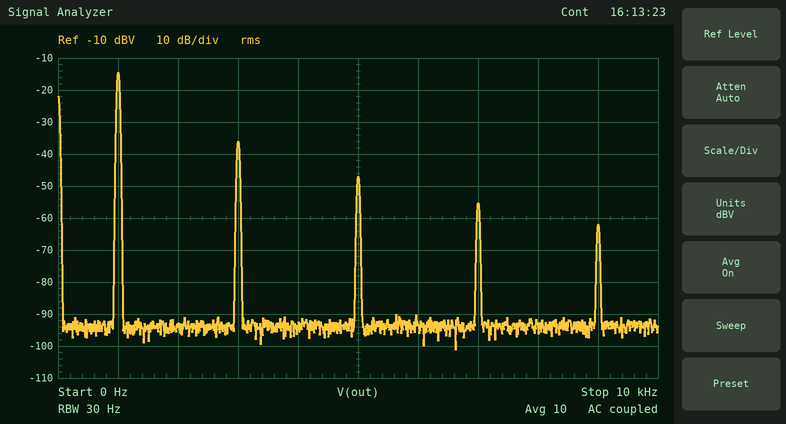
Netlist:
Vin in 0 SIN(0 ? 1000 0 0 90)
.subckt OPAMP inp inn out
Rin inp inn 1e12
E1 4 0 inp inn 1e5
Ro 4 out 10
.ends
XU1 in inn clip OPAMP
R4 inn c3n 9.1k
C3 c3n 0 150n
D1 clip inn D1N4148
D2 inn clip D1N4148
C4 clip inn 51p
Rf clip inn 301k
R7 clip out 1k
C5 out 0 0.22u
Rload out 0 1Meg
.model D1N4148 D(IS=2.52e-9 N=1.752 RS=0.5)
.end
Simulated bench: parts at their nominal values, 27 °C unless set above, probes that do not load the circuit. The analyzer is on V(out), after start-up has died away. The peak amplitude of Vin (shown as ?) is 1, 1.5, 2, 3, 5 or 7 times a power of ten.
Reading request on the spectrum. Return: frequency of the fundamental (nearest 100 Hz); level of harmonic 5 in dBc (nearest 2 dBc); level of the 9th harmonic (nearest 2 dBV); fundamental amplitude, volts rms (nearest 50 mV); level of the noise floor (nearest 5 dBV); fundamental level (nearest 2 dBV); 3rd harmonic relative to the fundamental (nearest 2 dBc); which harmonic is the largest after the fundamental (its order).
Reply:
1.0 kHz
-32 dBc
-62 dBV
200 mV
-95 dBV
-14 dBV
-22 dBc
3
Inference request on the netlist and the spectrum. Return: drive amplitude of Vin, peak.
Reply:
50 mV
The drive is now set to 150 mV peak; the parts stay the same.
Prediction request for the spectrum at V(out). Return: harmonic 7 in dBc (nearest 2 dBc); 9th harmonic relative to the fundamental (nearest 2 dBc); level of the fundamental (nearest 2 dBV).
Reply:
-38 dBc
-44 dBc
-12 dBV
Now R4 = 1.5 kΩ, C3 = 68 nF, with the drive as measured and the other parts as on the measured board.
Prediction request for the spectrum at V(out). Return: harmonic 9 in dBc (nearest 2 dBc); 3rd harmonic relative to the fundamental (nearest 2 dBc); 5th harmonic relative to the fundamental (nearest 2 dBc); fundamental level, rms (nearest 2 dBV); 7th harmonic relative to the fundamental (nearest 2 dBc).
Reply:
-42 dBc
-20 dBc
-30 dBc
-14 dBV
-36 dBc
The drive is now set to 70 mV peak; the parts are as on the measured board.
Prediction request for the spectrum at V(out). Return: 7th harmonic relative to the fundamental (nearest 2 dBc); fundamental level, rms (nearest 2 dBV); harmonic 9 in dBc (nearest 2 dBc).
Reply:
-40 dBc
-14 dBV
-46 dBc
